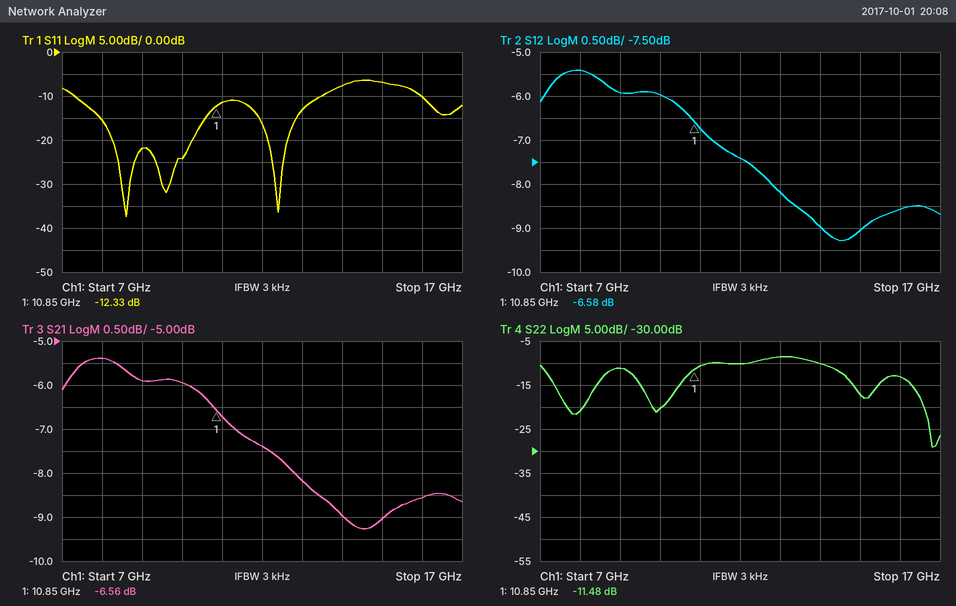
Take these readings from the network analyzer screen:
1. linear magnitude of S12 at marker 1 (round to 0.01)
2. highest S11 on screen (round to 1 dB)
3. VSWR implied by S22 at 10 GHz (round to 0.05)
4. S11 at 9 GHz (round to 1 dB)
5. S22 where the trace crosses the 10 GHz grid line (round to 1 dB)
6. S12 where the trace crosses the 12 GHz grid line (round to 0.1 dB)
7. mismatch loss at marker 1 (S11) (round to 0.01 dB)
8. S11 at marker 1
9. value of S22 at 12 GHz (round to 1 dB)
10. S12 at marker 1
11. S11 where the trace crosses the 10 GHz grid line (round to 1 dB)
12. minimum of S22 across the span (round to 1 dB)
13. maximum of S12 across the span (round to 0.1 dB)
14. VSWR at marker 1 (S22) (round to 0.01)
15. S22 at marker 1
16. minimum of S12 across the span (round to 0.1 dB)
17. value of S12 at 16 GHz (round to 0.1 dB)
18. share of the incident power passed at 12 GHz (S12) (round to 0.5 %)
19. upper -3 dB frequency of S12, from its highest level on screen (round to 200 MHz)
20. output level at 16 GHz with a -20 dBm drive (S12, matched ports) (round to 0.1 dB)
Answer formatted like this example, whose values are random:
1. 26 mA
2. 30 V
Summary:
1. 0.47
2. -6 dB
3. 1.20
4. -22 dB
5. -20 dB
6. -7.4 dB
7. 0.26 dB
8. -12.33 dB
9. -10 dB
10. -6.58 dB
11. -24 dB
12. -29 dB
13. -5.4 dB
14. 1.73
15. -11.48 dB
16. -9.3 dB
17. -8.6 dB
18. 18.0 %
19. 13.2 GHz
20. -28.6 dBm
